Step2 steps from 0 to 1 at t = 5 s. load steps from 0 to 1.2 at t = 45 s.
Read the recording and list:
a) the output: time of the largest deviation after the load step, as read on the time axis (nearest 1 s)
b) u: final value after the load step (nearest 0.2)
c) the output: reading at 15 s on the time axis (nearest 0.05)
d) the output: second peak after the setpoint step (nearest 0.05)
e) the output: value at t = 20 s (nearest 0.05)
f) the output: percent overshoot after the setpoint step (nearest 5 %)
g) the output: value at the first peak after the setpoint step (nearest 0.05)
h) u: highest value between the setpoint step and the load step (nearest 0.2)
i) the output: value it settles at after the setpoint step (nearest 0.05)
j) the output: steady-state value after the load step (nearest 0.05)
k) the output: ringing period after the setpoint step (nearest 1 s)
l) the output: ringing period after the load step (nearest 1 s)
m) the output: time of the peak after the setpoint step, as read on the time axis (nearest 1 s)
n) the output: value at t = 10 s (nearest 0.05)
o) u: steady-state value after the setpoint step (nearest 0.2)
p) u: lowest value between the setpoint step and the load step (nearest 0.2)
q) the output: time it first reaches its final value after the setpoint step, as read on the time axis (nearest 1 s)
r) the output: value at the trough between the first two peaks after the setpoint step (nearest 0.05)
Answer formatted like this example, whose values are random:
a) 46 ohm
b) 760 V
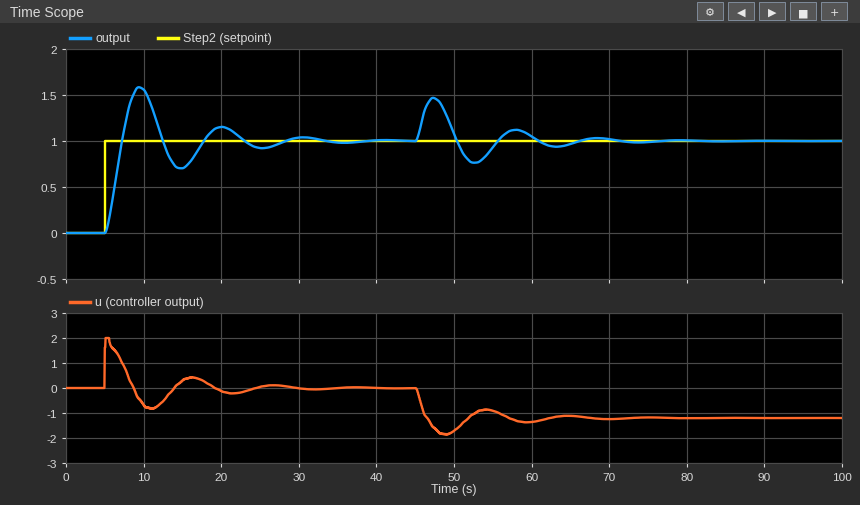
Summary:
a) 47 s
b) -1.2
c) 0.70
d) 1.15
e) 1.15
f) 60 %
g) 1.60
h) 2.0
i) 1.00
j) 1.00
k) 11 s
l) 11 s
m) 9 s
n) 1.55
o) 0.0
p) -0.8
q) 7 s
r) 0.70
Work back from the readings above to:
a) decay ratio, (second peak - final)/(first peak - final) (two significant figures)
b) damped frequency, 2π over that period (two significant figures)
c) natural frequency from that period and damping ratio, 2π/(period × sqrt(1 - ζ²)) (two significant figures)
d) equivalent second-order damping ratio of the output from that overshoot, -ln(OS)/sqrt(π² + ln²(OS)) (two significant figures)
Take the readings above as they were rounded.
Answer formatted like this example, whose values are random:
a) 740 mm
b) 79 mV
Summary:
a) 0.25
b) 0.57 rad/s
c) 0.58 rad/s
d) 0.16
